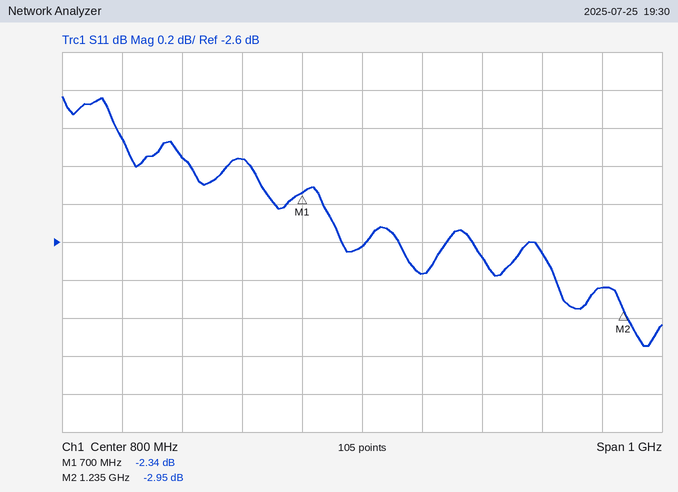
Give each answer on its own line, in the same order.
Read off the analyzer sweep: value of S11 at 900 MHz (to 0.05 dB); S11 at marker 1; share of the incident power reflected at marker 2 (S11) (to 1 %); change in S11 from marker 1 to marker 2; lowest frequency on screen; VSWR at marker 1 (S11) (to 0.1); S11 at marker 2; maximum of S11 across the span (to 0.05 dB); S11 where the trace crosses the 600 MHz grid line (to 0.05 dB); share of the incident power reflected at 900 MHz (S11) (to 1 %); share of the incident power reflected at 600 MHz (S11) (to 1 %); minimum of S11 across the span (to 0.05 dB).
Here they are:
-2.75 dB
-2.34 dB
51 %
-0.61 dB
300 MHz
7.5
-2.95 dB
-1.85 dB
-2.15 dB
53 %
61 %
-3.15 dB
